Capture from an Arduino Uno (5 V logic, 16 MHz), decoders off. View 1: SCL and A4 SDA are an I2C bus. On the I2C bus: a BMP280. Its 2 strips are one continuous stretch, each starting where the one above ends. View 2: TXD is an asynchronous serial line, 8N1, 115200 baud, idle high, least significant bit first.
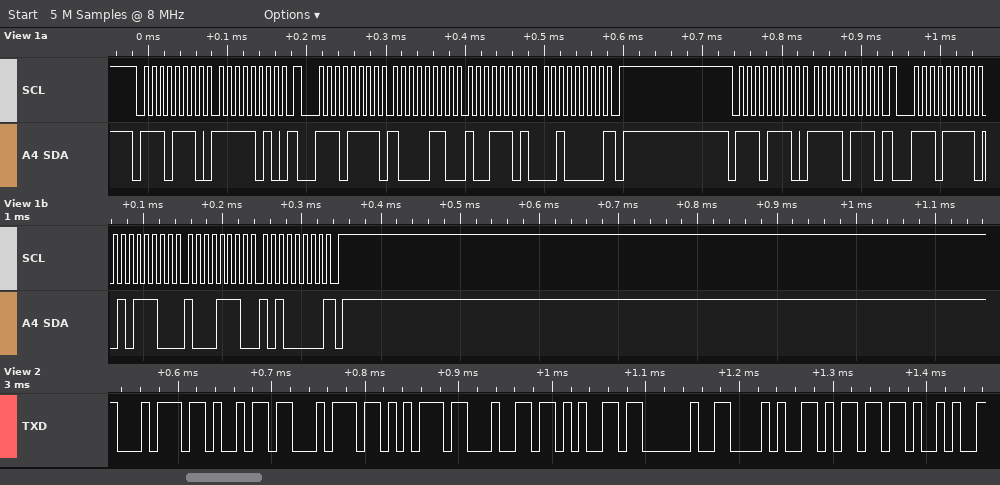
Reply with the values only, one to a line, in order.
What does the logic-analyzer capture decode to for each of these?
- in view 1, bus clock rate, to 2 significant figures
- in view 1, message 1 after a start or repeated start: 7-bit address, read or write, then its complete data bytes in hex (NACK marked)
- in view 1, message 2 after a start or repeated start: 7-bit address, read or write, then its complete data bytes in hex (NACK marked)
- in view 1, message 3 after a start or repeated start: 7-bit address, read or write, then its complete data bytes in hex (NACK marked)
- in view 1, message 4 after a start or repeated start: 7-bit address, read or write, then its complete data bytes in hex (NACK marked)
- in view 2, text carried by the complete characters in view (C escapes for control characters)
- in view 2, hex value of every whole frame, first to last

100 kHz
0x77 write: FA
0x77 read: 86 9D 20 NACK
0x77 write: F7
0x77 read: 5C 8E A0 NACK
"titude (m)"
74 69 74 75 64 65 20 28 6D 29
